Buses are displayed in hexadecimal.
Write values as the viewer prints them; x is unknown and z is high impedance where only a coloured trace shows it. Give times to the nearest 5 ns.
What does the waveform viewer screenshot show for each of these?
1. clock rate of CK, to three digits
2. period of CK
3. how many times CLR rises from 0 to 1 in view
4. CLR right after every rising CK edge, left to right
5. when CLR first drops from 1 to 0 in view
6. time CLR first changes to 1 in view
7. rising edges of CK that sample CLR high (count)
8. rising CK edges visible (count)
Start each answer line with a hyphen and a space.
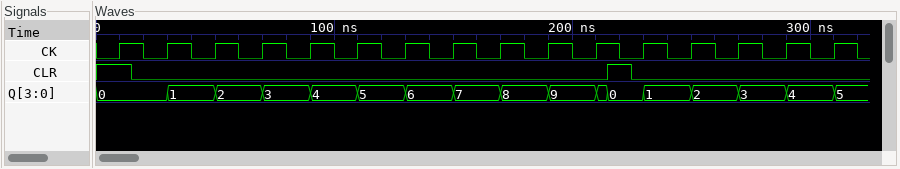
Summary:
- 50.0 MHz
- 20 ns
- 1
- 1 0 0 0 0 0 0 0 0 0 0 0 0 0 0 0
- 15 ns
- 215 ns
- 1
- 16
